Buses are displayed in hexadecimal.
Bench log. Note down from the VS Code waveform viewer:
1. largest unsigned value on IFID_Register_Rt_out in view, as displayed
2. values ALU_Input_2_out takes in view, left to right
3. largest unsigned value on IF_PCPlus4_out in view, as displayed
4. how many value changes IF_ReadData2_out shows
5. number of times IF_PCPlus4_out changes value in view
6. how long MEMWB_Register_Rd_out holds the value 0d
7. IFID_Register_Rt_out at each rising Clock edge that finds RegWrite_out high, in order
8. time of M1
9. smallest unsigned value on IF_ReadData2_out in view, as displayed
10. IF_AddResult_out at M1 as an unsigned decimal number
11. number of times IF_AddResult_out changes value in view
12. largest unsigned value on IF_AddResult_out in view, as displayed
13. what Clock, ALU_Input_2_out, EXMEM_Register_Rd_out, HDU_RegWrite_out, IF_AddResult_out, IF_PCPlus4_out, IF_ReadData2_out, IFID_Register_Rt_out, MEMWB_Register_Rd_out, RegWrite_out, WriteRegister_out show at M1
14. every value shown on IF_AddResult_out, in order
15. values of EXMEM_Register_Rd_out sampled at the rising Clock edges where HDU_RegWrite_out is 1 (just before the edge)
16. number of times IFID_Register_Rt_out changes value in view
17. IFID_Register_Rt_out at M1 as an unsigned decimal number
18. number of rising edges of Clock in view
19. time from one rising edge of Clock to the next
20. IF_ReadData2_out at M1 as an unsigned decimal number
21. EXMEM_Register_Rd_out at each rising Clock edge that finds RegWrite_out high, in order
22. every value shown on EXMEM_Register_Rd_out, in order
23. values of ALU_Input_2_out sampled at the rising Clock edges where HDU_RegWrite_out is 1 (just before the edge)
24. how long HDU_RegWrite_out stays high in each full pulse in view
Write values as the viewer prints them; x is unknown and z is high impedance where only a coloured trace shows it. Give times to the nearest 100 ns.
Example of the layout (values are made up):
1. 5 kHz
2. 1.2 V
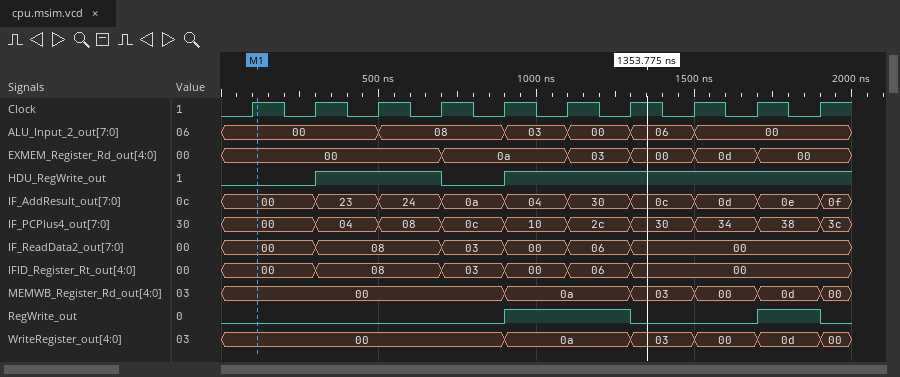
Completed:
1. 08
2. 00, 08, 03, 00, 06, 00
3. 3c
4. 5
5. 9
6. 200 ns
7. 00, 06, 00
8. 100 ns
9. 00
10. 0
11. 9
12. 30
13. Clock=1, ALU_Input_2_out=00, EXMEM_Register_Rd_out=00, HDU_RegWrite_out=0, IF_AddResult_out=00, IF_PCPlus4_out=00, IF_ReadData2_out=00, IFID_Register_Rt_out=00, MEMWB_Register_Rd_out=00, RegWrite_out=0, WriteRegister_out=00
14. 00, 23, 24, 0a, 04, 30, 0c, 0d, 0e, 0f
15. 00, 00, 0a, 03, 00, 0d, 00
16. 5
17. 0
18. 10
19. 200 ns
20. 0
21. 0a, 03, 00
22. 00, 0a, 03, 00, 0d, 00
23. 00, 08, 03, 00, 06, 00, 00
24. 400 ns
